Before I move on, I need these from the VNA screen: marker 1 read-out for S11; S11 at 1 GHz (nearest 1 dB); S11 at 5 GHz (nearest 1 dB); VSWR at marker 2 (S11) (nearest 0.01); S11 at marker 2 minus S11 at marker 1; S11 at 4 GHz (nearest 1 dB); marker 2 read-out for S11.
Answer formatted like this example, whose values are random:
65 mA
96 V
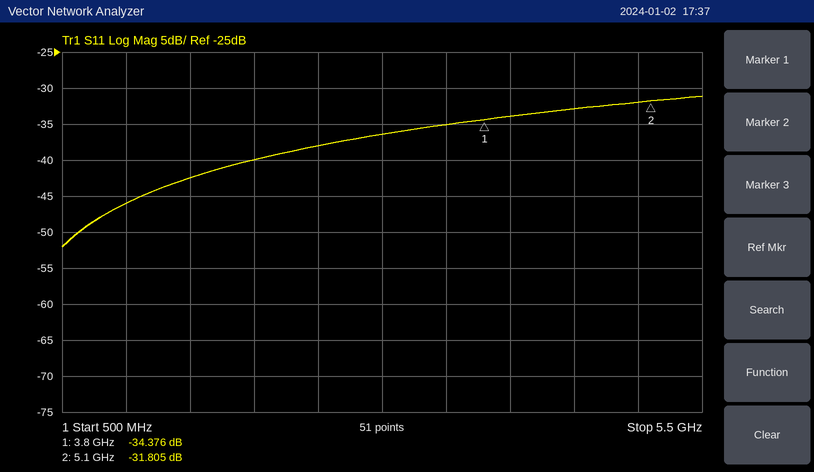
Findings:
-34.376 dB
-46 dB
-32 dB
1.05
2.571 dB
-34 dB
-31.805 dB
